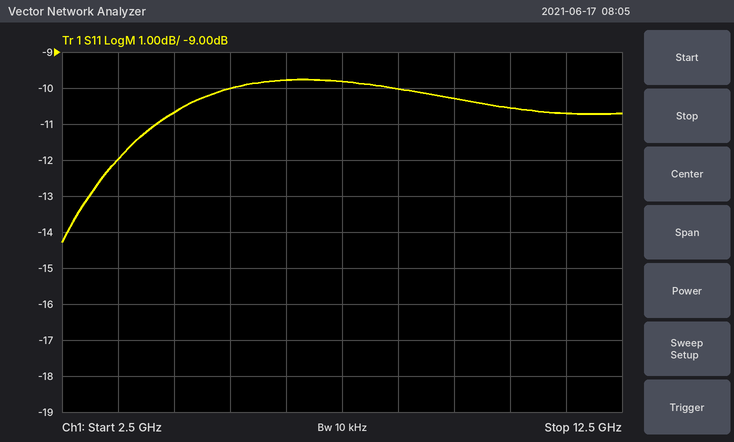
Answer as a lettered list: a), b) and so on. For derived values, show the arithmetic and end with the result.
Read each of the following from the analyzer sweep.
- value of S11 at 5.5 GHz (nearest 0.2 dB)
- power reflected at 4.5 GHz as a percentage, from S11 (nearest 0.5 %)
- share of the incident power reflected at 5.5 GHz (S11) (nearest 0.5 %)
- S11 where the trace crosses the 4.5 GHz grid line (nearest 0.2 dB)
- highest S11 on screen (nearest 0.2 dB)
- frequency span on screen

a) -10.0 dB
b) 10^(-10.6/10) ≈ 8.71 %, so 8.5 % to the nearest 0.5 %
c) 10^(-10/10) ≈ 10.0 %
d) -10.6 dB
e) -9.8 dB
f) 10 GHz
